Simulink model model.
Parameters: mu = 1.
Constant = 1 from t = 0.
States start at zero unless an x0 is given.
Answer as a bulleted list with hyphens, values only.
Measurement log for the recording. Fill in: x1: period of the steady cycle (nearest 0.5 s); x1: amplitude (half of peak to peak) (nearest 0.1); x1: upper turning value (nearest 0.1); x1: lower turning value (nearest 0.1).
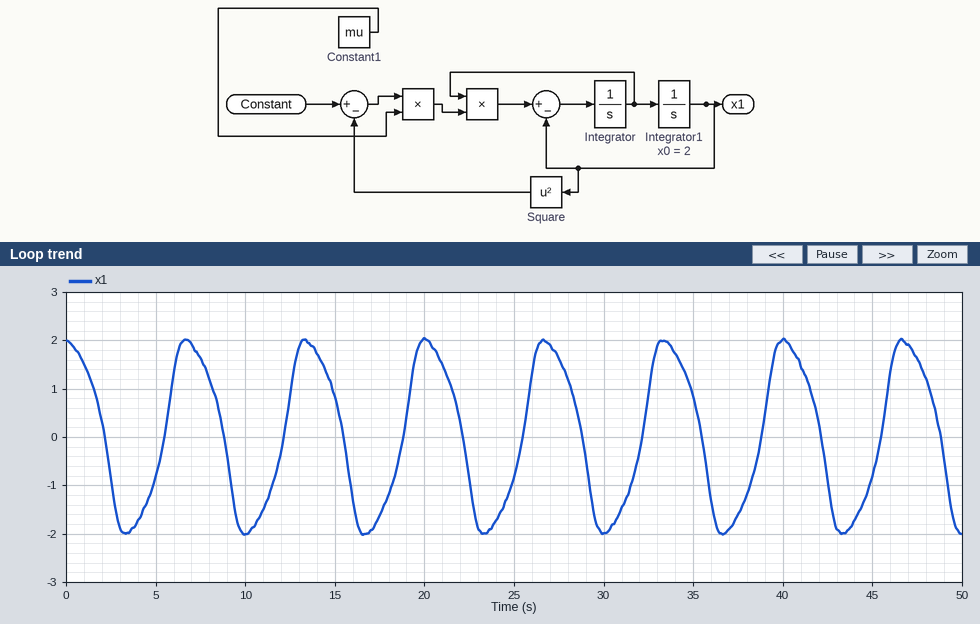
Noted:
- 6.5 s
- 2.0
- 2.0
- -2.0
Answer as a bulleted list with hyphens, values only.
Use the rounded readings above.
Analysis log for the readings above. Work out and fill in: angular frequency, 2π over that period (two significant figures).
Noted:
- 0.97 rad/s
